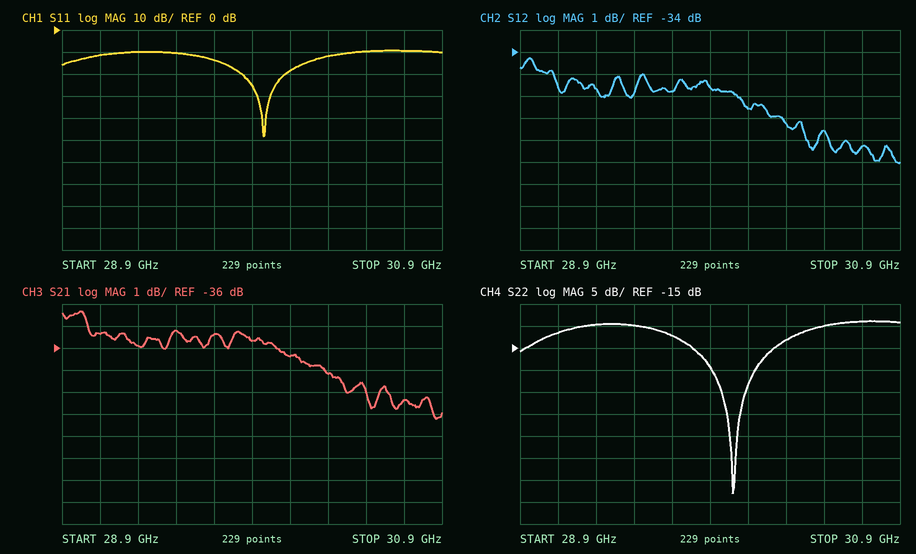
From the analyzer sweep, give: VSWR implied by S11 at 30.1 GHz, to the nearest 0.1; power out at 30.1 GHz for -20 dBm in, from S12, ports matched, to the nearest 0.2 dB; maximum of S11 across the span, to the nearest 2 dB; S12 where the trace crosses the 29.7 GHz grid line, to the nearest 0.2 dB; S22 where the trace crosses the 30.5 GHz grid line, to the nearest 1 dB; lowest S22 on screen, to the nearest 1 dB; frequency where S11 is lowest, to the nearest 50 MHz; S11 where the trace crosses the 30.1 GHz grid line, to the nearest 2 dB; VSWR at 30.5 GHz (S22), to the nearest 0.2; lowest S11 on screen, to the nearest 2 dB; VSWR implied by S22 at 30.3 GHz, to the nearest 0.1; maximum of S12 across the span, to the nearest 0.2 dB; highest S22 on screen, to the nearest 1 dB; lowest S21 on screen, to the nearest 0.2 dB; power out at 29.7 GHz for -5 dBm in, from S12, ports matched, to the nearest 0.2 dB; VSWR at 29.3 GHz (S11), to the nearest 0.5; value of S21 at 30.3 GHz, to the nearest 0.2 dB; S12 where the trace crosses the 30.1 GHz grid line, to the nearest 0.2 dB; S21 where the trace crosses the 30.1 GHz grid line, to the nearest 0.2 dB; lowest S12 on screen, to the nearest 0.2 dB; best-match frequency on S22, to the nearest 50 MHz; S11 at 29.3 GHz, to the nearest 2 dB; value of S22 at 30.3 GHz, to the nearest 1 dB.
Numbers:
1.3
-56.6 dBm
-10 dB
-35.8 dB
-10 dB
-48 dB
29.95 GHz
-18 dB
2.0
-48 dB
1.6
-34.2 dB
-9 dB
-39.2 dB
-40.8 dBm
2.0
-37.2 dB
-36.6 dB
-36.4 dB
-39.0 dB
30.00 GHz
-10 dB
-13 dB
